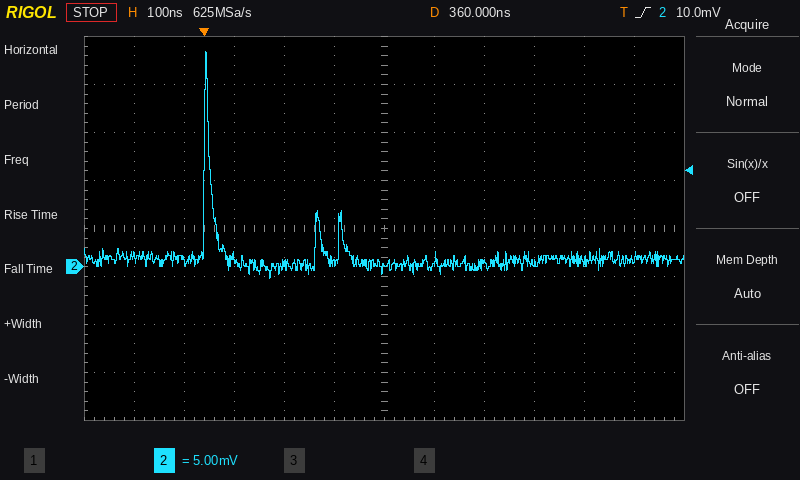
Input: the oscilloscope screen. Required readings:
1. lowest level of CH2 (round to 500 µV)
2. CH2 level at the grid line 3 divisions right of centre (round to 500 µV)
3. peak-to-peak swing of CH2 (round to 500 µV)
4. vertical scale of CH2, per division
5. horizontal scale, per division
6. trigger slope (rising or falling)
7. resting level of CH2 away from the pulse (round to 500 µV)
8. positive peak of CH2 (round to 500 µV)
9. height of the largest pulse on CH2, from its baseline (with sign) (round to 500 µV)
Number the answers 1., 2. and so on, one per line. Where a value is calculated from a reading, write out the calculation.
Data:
1. -1.0 mV
2. 500 µV
3. 22.5 mV − (-1.0 mV) = 23.5 mV
4. 5 mV
5. 100 ns
6. rising
7. 500 µV
8. 22.5 mV
9. 22.5 mV − (500 µV) = +22.0 mV
